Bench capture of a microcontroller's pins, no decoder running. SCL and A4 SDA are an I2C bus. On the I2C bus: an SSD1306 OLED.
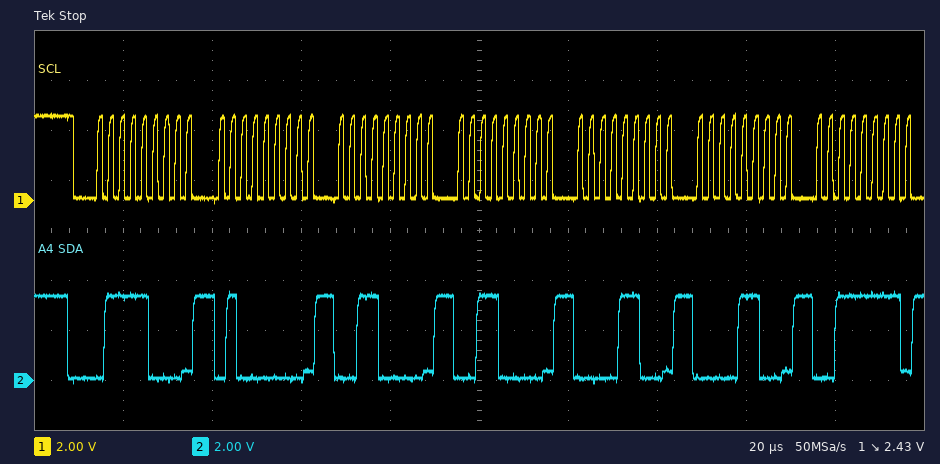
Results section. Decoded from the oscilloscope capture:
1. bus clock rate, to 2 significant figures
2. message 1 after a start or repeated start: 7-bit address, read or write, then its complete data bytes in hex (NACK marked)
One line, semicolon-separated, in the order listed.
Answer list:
400 kHz; 0x3C write: 40 30 30 0C 0C 3F
